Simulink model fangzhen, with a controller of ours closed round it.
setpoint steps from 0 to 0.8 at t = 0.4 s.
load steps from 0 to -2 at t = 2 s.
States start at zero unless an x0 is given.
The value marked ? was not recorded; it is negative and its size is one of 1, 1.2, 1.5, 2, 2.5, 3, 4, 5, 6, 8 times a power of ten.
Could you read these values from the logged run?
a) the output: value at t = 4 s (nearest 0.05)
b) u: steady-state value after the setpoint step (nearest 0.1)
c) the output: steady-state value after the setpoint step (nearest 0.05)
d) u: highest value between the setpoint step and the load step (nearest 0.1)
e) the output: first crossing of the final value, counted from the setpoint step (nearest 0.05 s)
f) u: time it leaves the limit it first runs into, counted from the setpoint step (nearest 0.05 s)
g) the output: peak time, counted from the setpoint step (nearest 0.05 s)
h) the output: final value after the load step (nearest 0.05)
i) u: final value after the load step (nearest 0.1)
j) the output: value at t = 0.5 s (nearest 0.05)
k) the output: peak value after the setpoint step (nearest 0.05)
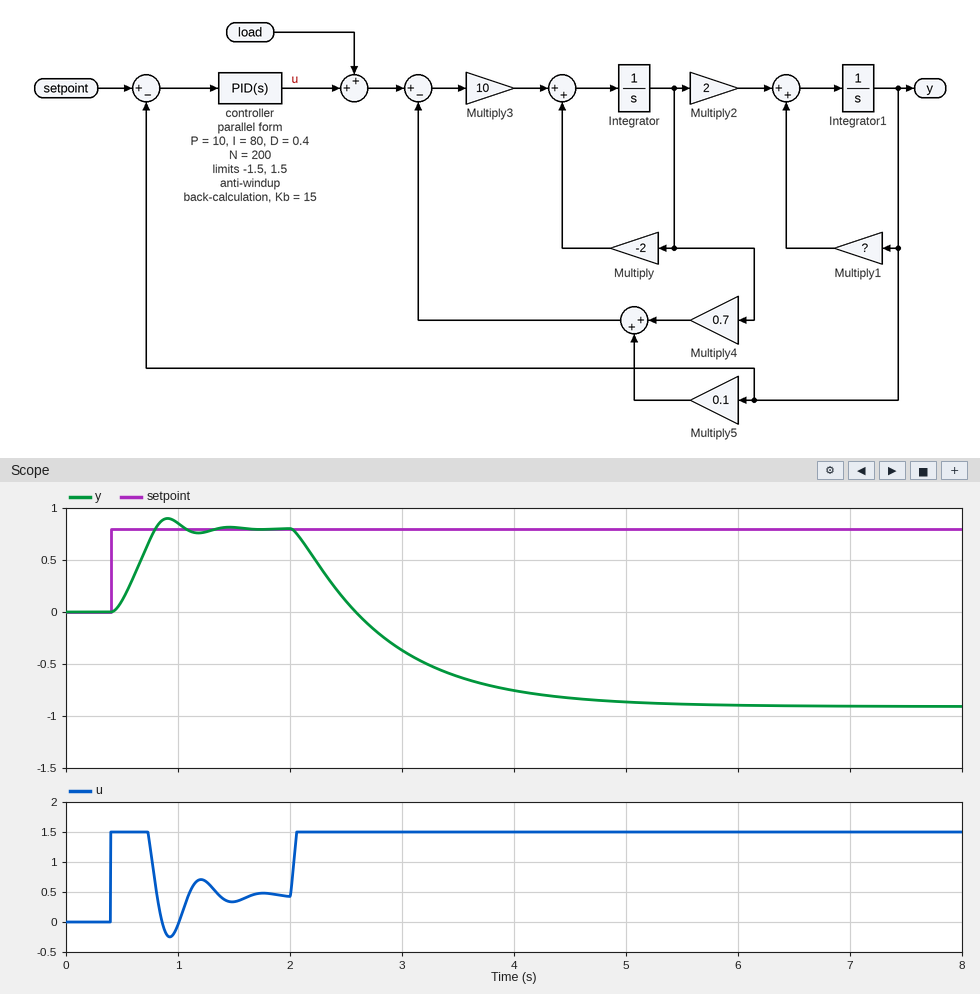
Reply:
-0.75
0.4
0.80
1.5
0.40 s
0.35 s
0.50 s
-0.90
1.5
0.10
0.90
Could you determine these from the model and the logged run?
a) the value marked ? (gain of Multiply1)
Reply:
-1
